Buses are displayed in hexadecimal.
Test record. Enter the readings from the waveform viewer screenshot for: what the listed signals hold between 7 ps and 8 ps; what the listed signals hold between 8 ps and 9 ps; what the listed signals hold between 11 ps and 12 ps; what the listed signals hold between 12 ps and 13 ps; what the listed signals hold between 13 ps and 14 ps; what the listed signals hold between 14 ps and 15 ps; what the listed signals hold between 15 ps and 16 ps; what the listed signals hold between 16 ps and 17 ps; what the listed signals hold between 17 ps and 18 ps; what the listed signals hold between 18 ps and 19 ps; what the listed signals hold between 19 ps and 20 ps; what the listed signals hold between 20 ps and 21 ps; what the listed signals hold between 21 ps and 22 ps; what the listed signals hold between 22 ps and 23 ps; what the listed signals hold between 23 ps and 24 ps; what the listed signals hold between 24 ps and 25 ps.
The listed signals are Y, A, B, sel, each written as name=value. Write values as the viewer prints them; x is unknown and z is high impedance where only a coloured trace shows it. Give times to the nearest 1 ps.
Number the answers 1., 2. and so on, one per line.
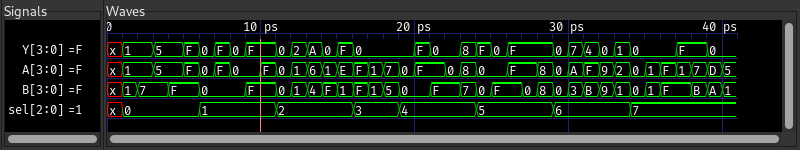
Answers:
1. Y=F, A=F, B=0, sel=1
2. Y=0, A=0, B=0, sel=1
3. Y=0, A=0, B=0, sel=2
4. Y=2, A=1, B=1, sel=2
5. Y=A, A=6, B=4, sel=2
6. Y=0, A=1, B=F, sel=2
7. Y=F, A=E, B=1, sel=2
8. Y=0, A=F, B=F, sel=3
9. Y=0, A=1, B=1, sel=3
10. Y=0, A=7, B=5, sel=3
11. Y=0, A=0, B=0, sel=4
12. Y=F, A=F, B=0, sel=4
13. Y=0, A=F, B=F, sel=4
14. Y=0, A=0, B=F, sel=4
15. Y=8, A=8, B=7, sel=4
16. Y=F, A=0, B=0, sel=5
